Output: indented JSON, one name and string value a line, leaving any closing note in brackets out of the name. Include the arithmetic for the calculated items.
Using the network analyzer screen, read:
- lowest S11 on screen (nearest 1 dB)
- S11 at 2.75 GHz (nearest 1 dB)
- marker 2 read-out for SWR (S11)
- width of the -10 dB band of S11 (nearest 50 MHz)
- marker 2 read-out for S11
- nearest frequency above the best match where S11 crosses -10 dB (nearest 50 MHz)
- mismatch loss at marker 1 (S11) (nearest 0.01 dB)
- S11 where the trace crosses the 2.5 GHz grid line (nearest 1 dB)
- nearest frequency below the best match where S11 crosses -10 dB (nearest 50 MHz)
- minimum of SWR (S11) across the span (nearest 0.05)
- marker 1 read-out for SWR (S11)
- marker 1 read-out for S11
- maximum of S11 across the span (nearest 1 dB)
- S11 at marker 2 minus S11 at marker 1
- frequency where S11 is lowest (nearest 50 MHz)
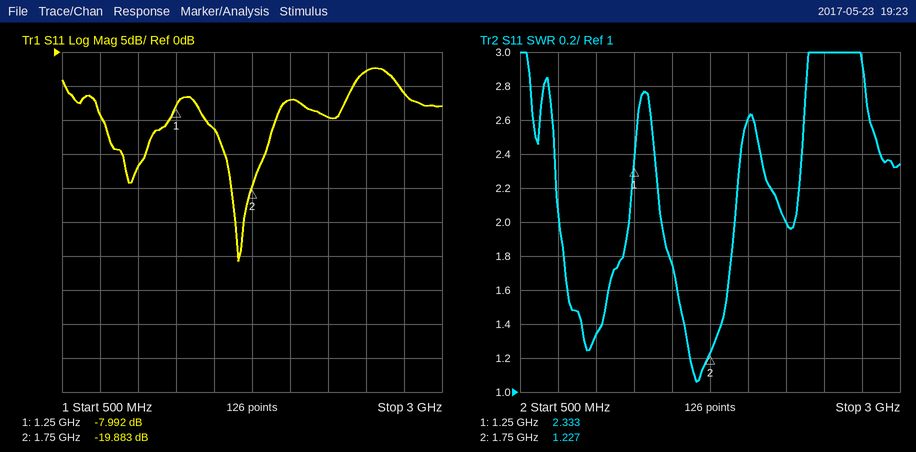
{
  "lowest S11 on screen": "-31 dB",
  "S11 at 2.75 GHz": "-6 dB",
  "marker 2 read-out for SWR": "1.227",
  "width of the -10 dB band of S11": "1.90 GHz − 1.45 GHz = 450 MHz",
  "marker 2 read-out for S11": "-19.883 dB",
  "nearest frequency above the best match where S11 crosses -10 dB": "1.90 GHz",
  "mismatch loss at marker 1 (S11)": "−10 log10(1 − 10^(-7.992/10)) ≈ 0.75 dB",
  "S11 where the trace crosses the 2.5 GHz grid line": "-3 dB",
  "nearest frequency below the best match where S11 crosses -10 dB": "1.45 GHz",
  "minimum of SWR (S11) across the span": "1.05",
  "marker 1 read-out for SWR": "2.333",
  "marker 1 read-out for S11": "-7.992 dB",
  "maximum of S11 across the span": "-2 dB",
  "S11 at marker 2 minus S11 at marker 1": "-19.883 − (-7.992) = -11.891 dB",
  "frequency where S11 is lowest": "1.65 GHz"
}
